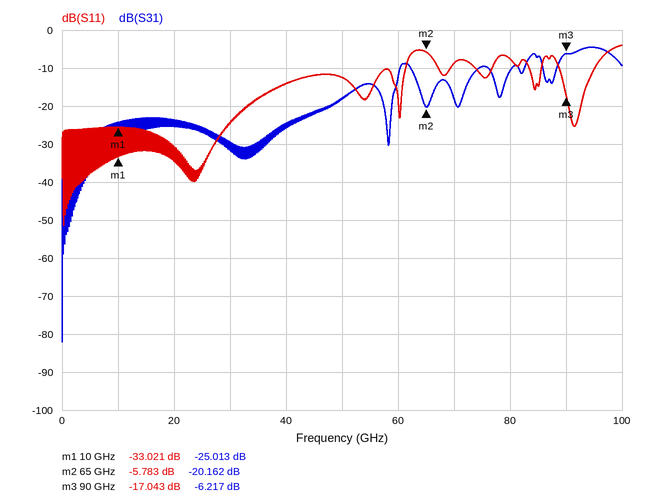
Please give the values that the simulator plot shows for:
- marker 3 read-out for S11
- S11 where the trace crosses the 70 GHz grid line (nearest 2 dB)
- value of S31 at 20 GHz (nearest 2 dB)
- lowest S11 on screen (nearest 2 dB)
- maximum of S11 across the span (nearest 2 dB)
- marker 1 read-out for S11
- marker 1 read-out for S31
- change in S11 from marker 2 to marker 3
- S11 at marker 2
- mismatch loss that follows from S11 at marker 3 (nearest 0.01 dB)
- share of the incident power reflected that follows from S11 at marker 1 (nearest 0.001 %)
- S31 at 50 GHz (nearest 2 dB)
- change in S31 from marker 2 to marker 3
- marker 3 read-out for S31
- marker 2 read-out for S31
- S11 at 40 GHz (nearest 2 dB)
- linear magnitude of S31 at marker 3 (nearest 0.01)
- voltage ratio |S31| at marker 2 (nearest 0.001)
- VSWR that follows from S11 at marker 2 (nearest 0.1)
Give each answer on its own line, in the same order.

-17.043 dB
-8 dB
-24 dB
-52 dB
-4 dB
-33.021 dB
-25.013 dB
-11.260 dB
-5.783 dB
0.09 dB
0.050 %
-18 dB
13.945 dB
-6.217 dB
-20.162 dB
-14 dB
0.49
0.098
3.1
